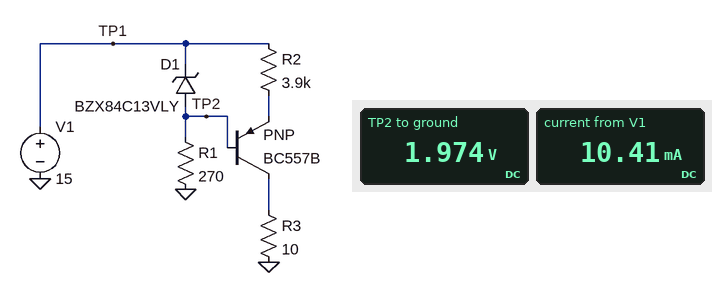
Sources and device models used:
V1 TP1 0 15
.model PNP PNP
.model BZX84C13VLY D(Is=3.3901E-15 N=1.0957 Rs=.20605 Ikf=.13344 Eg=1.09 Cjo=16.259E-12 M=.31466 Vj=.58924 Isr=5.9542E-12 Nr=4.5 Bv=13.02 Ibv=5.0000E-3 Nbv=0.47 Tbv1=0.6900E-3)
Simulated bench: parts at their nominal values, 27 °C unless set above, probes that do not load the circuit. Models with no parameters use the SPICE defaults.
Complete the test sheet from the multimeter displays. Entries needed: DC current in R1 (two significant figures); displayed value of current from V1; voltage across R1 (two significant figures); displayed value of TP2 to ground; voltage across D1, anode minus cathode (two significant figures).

7.3 mA
10.41 mA
2.0 V
1.974 V
-13 V
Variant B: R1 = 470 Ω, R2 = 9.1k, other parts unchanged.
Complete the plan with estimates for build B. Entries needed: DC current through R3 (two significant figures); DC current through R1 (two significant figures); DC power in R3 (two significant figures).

1.3 mA
4.2 mA
18 µW
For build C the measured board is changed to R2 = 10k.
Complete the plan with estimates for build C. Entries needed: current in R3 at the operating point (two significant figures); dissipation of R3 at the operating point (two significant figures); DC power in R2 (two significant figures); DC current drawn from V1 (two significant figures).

1.2 mA
15 µW
15 mW
8.5 mA
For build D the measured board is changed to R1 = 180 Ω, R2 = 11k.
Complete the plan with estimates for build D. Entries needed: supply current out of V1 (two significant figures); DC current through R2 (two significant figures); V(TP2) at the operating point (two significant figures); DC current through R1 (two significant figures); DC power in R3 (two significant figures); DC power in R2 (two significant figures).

12 mA
1.1 mA
2.0 V
11 mA
12 µW
14 mW
